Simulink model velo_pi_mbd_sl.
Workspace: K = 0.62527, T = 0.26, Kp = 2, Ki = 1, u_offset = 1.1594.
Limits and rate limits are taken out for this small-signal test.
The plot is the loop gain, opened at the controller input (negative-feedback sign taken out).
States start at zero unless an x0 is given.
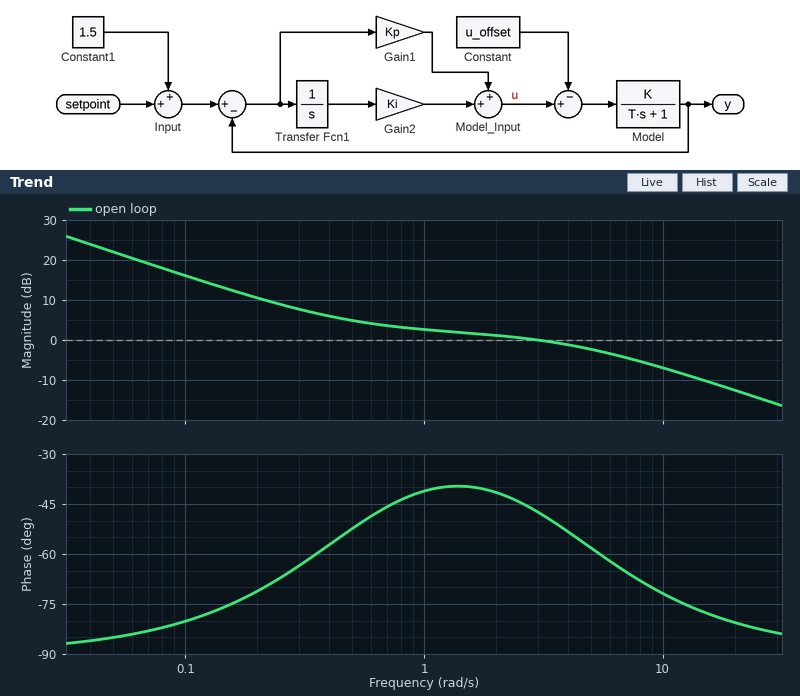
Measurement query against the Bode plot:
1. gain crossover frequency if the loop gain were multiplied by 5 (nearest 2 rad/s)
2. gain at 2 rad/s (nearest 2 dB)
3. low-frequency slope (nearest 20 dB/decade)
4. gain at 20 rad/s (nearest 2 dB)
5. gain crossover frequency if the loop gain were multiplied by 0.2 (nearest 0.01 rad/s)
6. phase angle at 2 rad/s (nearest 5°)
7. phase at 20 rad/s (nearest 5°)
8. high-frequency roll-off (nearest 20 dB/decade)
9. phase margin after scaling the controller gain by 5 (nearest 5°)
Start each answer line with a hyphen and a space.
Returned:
- 24 rad/s
- 2 dB
- -20 dB/decade
- -12 dB
- 0.13 rad/s
- -40°
- -80°
- -20 dB/decade
- 100°
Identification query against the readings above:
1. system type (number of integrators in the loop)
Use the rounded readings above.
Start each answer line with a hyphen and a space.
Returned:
- 1
